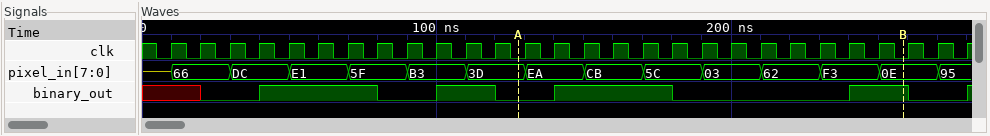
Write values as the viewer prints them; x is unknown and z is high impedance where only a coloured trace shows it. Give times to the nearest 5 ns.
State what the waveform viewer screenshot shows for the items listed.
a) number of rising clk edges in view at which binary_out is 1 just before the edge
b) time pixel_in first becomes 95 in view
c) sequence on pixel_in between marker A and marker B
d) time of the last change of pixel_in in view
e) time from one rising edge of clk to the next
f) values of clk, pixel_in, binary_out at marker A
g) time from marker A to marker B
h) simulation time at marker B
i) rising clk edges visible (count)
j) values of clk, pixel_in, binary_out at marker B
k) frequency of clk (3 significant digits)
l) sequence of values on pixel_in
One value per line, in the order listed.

12
270 ns
3D, EA, CB, 5C, 03, 62, F3, 0E
270 ns
10 ns
clk=0, pixel_in=3D, binary_out=0
130 ns
260 ns
28
clk=0, pixel_in=0E, binary_out=1
100 MHz
z, 66, DC, E1, 5F, B3, 3D, EA, CB, 5C, 03, 62, F3, 0E, 95
